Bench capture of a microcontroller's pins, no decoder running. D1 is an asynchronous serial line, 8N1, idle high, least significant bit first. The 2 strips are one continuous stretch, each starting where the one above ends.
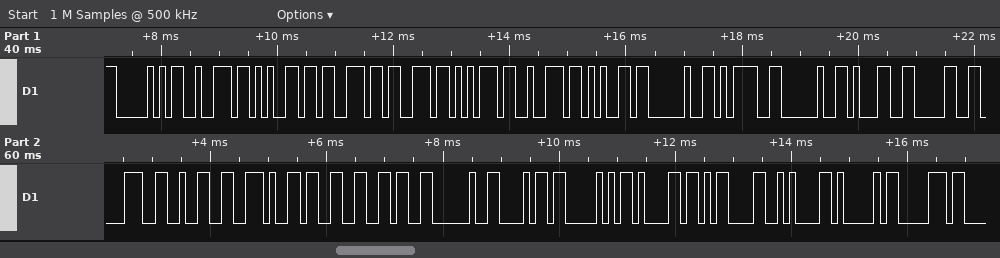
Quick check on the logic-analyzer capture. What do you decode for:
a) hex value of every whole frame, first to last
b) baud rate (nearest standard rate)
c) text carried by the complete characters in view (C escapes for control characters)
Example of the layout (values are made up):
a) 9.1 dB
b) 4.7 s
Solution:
a) 50 72 65 73 73 75 72 65 20 3D 20 31 30 38 32 2E 33 36 20 68 50 61 0D 0A 41 70
b) 9600 baud
c) "Pressure = 1082.36 hPa\r\nAp"
